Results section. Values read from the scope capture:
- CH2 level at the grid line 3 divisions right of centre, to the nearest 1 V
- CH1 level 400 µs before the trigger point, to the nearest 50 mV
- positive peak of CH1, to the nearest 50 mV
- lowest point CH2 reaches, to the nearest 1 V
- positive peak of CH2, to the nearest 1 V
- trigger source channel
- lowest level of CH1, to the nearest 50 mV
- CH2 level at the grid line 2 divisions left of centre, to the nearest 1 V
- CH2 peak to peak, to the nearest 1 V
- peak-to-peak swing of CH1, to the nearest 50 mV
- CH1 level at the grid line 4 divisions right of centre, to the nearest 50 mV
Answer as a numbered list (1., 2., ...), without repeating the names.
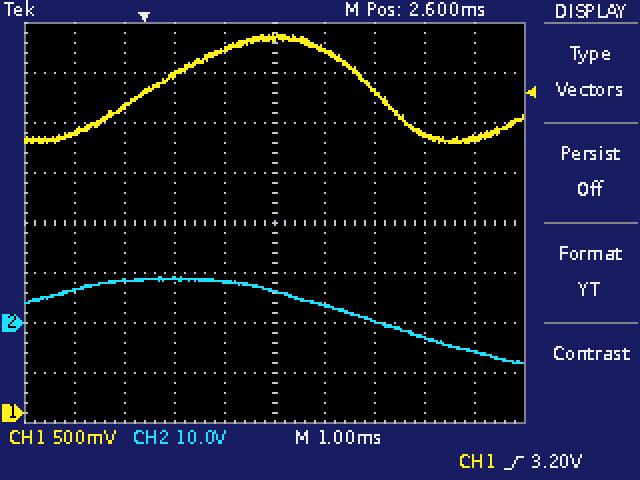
1. -3 V
2. 3.05 V
3. 3.80 V
4. -8 V
5. 9 V
6. CH1
7. 2.70 V
8. 9 V
9. 17 V
10. 1.10 V
11. 2.75 V
